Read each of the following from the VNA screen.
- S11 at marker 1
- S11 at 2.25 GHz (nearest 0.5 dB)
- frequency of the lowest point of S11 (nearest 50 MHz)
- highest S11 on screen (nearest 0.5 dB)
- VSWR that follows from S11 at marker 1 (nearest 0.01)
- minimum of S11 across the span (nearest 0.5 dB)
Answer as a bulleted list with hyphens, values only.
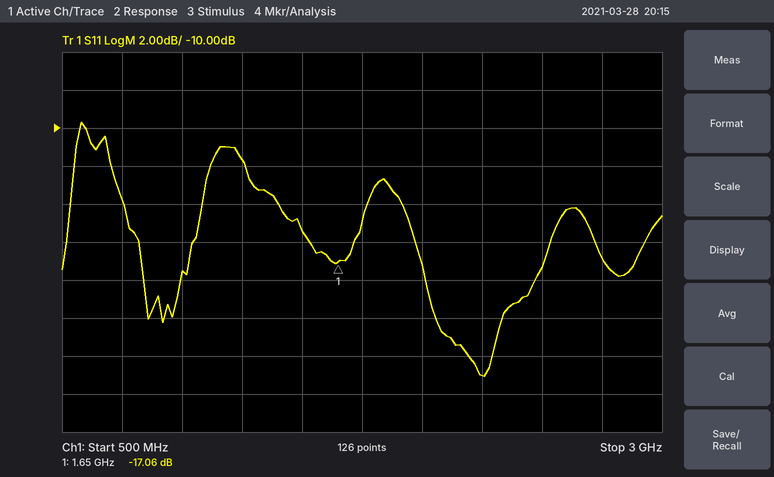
- -17.06 dB
- -23.0 dB
- 2.25 GHz
- -9.5 dB
- 1.33
- -23.0 dB
